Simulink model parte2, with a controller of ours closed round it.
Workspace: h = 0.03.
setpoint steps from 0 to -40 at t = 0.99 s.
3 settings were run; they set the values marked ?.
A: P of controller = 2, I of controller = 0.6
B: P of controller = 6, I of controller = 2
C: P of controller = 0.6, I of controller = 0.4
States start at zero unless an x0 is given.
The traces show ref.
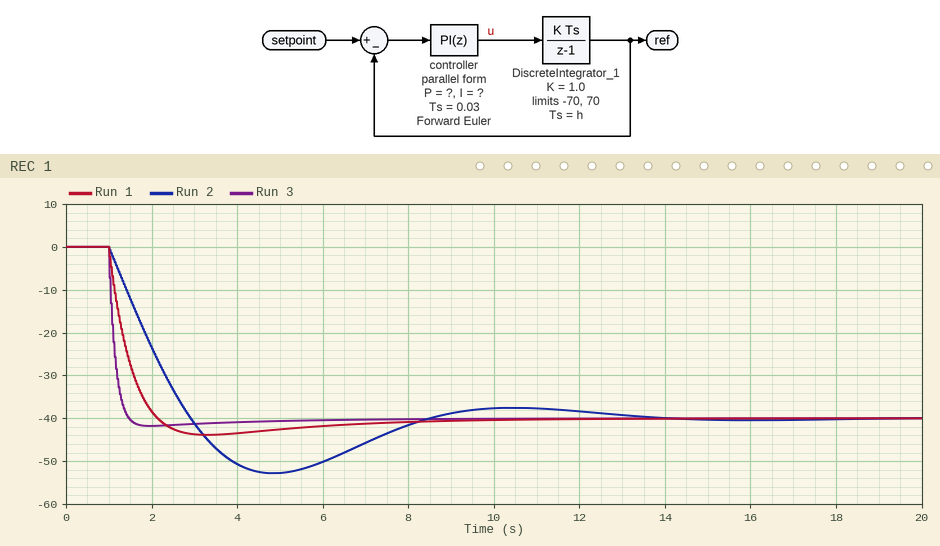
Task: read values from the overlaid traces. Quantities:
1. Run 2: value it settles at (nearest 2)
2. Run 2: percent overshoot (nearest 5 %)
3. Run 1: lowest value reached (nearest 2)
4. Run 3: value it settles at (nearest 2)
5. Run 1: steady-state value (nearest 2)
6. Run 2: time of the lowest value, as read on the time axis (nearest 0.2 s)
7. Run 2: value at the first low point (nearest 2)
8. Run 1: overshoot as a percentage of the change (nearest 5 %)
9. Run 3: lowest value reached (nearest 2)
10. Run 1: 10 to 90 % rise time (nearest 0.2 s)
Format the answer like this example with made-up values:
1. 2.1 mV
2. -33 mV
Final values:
1. -40
2. 30 %
3. -44
4. -40
5. -40
6. 4.8 s
7. -52
8. 10 %
9. -42
10. 0.8 s
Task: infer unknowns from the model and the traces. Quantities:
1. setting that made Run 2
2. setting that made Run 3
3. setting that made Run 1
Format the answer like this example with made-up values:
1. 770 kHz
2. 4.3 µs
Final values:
1. C
2. B
3. A
